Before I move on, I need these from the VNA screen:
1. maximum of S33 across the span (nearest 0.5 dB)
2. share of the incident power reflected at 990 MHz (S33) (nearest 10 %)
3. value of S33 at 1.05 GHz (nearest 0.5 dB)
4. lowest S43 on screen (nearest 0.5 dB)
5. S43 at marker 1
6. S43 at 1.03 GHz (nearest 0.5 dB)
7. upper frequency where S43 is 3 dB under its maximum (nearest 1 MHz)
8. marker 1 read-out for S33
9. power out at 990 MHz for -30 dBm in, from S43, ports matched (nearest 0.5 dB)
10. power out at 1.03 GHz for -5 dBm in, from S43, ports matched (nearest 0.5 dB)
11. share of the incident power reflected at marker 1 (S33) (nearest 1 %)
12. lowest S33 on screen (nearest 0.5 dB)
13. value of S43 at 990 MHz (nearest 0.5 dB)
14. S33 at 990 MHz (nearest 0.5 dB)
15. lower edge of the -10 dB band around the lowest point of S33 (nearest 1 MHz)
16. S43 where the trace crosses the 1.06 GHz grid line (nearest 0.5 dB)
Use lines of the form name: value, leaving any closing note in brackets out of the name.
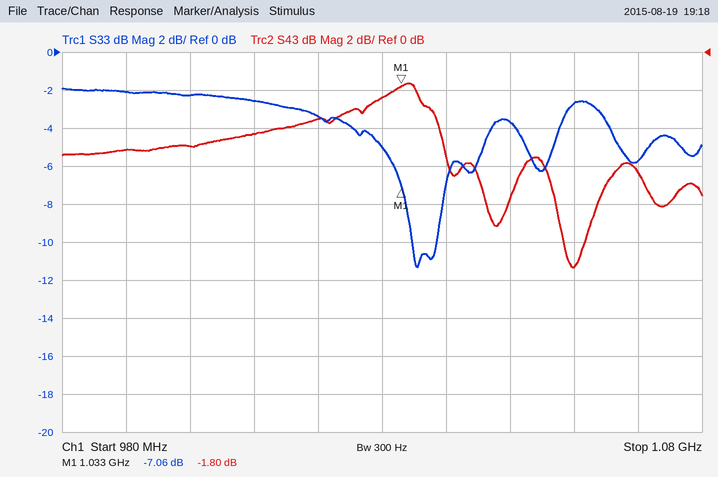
maximum of S33 across the span: -2.0 dB
share of the incident power reflected at 990 MHz (S33): 60 %
value of S33 at 1.05 GHz: -3.5 dB
lowest S43 on screen: -11.5 dB
S43 at marker 1: -1.80 dB
S43 at 1.03 GHz: -2.5 dB
upper frequency where S43 is 3 dB under its maximum: 1.039 GHz
marker 1 read-out for S33: -7.06 dB
power out at 990 MHz for -30 dBm in, from S43, ports matched: -35.0 dBm
power out at 1.03 GHz for -5 dBm in, from S43, ports matched: -7.5 dBm
share of the incident power reflected at marker 1 (S33): 20 %
lowest S33 on screen: -11.5 dB
value of S43 at 990 MHz: -5.0 dB
S33 at 990 MHz: -2.0 dB
lower edge of the -10 dB band around the lowest point of S33: 1.035 GHz
S43 where the trace crosses the 1.06 GHz grid line: -11.5 dB
